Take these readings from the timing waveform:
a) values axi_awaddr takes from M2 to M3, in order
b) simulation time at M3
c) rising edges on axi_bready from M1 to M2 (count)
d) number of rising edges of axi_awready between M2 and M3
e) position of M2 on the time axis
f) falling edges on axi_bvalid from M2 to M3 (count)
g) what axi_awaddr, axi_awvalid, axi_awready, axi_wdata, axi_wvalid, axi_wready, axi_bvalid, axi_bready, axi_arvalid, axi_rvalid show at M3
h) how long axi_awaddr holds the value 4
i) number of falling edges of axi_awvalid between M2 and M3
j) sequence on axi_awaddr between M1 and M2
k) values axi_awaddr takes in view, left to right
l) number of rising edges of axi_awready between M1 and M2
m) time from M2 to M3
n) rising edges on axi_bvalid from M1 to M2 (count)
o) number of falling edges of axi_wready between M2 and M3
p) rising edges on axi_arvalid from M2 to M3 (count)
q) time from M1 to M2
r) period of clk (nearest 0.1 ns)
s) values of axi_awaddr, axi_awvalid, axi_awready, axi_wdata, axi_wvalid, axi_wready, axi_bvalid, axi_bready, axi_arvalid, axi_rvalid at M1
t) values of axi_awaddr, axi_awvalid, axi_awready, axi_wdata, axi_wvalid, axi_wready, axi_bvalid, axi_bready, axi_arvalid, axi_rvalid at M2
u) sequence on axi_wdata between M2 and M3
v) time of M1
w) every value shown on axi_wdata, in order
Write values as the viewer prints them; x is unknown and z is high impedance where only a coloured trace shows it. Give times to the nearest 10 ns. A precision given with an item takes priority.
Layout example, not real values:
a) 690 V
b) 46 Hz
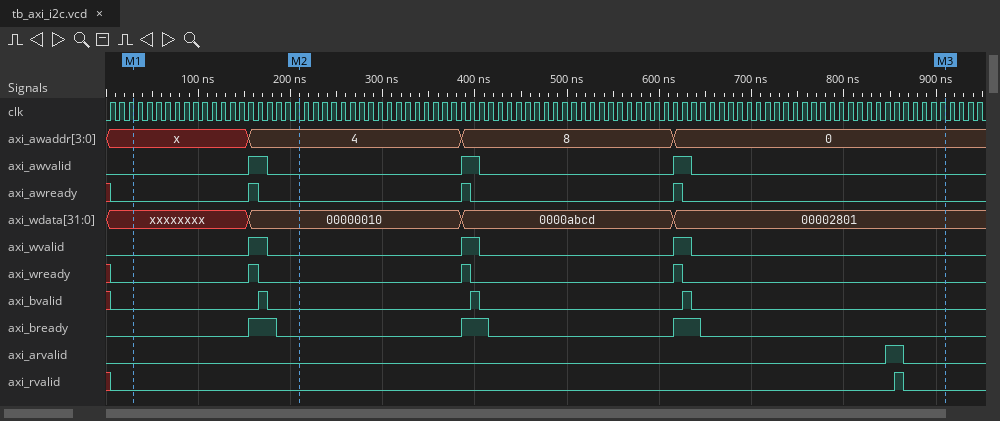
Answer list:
a) 4, 8, 0
b) 910 ns
c) 1
d) 2
e) 210 ns
f) 2
g) axi_awaddr=0, axi_awvalid=0, axi_awready=0, axi_wdata=00002801, axi_wvalid=0, axi_wready=0, axi_bvalid=0, axi_bready=0, axi_arvalid=0, axi_rvalid=0
h) 230 ns
i) 2
j) x, 4
k) x, 4, 8, 0
l) 1
m) 700 ns
n) 1
o) 2
p) 1
q) 180 ns
r) 10 ns
s) axi_awaddr=x, axi_awvalid=0, axi_awready=0, axi_wdata=xxxxxxxx, axi_wvalid=0, axi_wready=0, axi_bvalid=0, axi_bready=0, axi_arvalid=0, axi_rvalid=0
t) axi_awaddr=4, axi_awvalid=0, axi_awready=0, axi_wdata=00000010, axi_wvalid=0, axi_wready=0, axi_bvalid=0, axi_bready=0, axi_arvalid=0, axi_rvalid=0
u) 00000010, 0000abcd, 00002801
v) 30 ns
w) xxxxxxxx, 00000010, 0000abcd, 00002801
